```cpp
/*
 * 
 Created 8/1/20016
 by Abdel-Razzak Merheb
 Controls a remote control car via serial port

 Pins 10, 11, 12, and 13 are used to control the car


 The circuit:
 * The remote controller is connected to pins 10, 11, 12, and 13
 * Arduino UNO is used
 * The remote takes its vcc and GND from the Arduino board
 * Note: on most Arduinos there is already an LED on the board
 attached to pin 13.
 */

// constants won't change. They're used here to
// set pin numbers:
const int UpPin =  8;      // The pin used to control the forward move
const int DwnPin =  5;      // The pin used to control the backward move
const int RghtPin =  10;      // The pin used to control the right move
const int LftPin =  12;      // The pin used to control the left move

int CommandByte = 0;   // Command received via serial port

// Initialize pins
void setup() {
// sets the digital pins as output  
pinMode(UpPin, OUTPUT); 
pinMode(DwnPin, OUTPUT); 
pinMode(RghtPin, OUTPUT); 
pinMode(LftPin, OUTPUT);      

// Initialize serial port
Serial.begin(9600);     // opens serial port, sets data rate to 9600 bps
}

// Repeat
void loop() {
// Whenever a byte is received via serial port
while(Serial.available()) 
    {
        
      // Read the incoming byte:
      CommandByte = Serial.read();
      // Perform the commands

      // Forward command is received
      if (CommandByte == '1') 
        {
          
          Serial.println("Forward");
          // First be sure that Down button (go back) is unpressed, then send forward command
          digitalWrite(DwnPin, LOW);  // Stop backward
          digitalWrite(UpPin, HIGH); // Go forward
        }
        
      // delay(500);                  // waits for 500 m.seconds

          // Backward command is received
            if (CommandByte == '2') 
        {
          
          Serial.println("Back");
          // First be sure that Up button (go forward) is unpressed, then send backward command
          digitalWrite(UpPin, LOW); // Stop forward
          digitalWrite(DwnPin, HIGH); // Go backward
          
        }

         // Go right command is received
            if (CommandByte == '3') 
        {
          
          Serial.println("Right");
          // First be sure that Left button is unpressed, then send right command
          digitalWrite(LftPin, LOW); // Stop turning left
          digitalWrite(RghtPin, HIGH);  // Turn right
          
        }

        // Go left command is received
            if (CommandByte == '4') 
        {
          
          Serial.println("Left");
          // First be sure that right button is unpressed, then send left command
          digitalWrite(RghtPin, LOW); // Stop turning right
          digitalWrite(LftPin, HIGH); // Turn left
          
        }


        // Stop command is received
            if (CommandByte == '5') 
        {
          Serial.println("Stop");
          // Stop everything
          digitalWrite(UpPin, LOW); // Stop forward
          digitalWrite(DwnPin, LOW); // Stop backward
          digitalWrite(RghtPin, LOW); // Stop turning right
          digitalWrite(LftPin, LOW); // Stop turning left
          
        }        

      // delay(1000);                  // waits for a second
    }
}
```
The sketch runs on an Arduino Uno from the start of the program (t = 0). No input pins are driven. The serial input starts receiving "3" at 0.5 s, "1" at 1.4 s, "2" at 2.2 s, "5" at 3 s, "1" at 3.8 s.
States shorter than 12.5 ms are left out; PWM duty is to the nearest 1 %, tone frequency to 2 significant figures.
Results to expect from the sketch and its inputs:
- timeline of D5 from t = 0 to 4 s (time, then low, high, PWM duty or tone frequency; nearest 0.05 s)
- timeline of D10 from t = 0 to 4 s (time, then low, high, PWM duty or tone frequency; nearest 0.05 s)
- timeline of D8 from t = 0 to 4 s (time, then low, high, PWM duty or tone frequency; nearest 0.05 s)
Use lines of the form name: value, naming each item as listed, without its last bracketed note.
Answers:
timeline of D5 from t = 0 to 4 s: 0 s low; 2.2 s high; 3 s low
timeline of D10 from t = 0 to 4 s: 0 s low; 0.5 s high; 3 s low
timeline of D8 from t = 0 to 4 s: 0 s low; 1.4 s high; 2.2 s low; 3.8 s high
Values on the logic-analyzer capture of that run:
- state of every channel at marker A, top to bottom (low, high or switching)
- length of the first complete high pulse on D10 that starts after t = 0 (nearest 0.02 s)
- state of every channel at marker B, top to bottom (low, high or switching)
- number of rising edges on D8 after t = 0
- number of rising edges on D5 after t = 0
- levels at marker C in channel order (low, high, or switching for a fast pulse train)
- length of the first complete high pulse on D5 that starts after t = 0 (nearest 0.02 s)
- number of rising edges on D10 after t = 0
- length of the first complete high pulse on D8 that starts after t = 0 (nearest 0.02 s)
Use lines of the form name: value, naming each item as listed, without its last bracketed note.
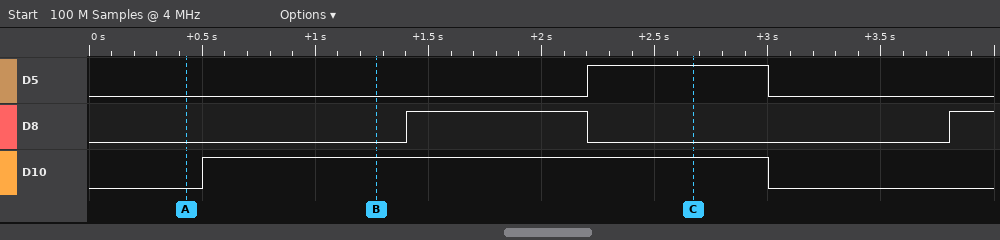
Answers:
state of every channel at marker A, top to bottom: D5 low, D8 low, D10 low
length of the first complete high pulse on D10 that starts after t = 0: 2.50 s
state of every channel at marker B, top to bottom: D5 low, D8 low, D10 high
number of rising edges on D8 after t = 0: 2
number of rising edges on D5 after t = 0: 1
levels at marker C in channel order: D5 high, D8 low, D10 high
length of the first complete high pulse on D5 that starts after t = 0: 0.80 s
number of rising edges on D10 after t = 0: 1
length of the first complete high pulse on D8 that starts after t = 0: 0.80 s
